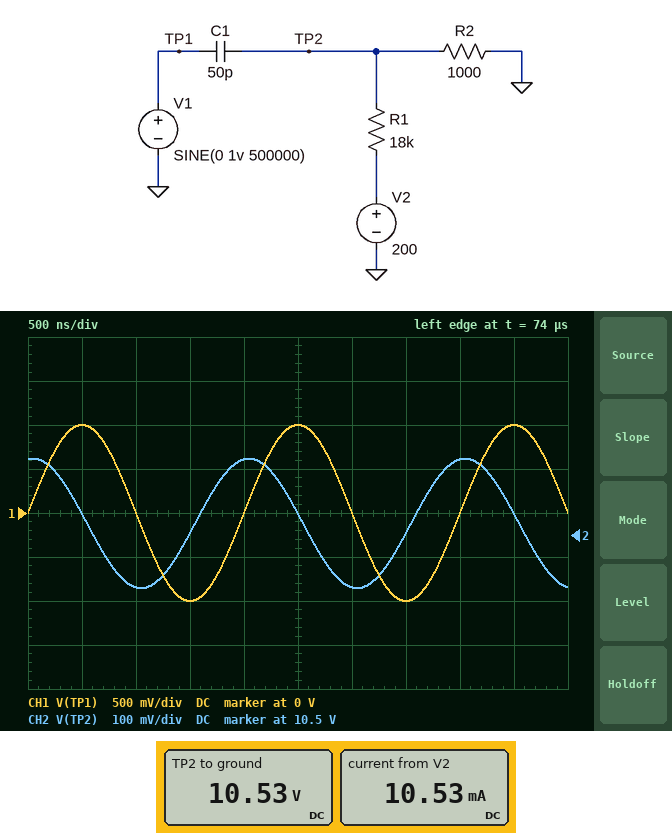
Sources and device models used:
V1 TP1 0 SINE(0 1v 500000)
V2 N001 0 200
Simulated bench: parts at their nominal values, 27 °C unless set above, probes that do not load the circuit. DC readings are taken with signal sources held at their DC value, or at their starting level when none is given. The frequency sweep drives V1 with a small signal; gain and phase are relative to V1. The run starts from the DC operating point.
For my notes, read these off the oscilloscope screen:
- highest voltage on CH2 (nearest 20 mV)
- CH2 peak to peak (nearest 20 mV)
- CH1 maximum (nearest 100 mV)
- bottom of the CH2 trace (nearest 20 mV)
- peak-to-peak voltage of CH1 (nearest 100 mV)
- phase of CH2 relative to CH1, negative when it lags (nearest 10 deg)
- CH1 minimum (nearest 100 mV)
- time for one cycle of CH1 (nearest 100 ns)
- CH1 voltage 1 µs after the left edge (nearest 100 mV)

10.68 V
300 mV
1.0 V
10.38 V
2.0 V
80 deg
-1.0 V
2.0 µs
0 V
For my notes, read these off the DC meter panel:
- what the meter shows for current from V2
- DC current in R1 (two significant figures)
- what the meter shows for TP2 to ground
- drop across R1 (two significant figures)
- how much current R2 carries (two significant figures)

10.53 mA
11 mA
10.53 V
190 V
11 mA
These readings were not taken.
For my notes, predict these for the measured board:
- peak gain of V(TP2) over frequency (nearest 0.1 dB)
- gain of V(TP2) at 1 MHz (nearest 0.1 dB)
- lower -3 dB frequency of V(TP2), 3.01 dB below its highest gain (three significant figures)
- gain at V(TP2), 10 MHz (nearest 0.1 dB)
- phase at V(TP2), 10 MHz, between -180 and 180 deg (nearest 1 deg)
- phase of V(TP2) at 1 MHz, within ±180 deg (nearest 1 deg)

0 dB
-10.9 dB
3.36 MHz
-0.5 dB
19 deg
73 deg
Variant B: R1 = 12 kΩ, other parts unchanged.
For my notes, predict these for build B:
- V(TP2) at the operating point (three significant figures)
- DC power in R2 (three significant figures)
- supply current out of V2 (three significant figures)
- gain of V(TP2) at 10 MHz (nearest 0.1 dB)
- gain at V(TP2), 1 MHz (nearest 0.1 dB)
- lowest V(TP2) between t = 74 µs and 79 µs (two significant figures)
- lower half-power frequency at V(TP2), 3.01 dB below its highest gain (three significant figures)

15.4 V
237 mW
15.4 mA
-0.5 dB
-11.1 dB
15 V
3.45 MHz
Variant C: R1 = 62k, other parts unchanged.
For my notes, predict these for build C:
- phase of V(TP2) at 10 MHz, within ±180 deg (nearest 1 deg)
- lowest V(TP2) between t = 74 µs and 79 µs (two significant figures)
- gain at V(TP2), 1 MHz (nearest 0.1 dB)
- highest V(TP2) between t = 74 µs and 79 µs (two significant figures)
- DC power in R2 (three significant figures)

18 deg
3.0 V
-10.6 dB
3.3 V
10.1 mW
